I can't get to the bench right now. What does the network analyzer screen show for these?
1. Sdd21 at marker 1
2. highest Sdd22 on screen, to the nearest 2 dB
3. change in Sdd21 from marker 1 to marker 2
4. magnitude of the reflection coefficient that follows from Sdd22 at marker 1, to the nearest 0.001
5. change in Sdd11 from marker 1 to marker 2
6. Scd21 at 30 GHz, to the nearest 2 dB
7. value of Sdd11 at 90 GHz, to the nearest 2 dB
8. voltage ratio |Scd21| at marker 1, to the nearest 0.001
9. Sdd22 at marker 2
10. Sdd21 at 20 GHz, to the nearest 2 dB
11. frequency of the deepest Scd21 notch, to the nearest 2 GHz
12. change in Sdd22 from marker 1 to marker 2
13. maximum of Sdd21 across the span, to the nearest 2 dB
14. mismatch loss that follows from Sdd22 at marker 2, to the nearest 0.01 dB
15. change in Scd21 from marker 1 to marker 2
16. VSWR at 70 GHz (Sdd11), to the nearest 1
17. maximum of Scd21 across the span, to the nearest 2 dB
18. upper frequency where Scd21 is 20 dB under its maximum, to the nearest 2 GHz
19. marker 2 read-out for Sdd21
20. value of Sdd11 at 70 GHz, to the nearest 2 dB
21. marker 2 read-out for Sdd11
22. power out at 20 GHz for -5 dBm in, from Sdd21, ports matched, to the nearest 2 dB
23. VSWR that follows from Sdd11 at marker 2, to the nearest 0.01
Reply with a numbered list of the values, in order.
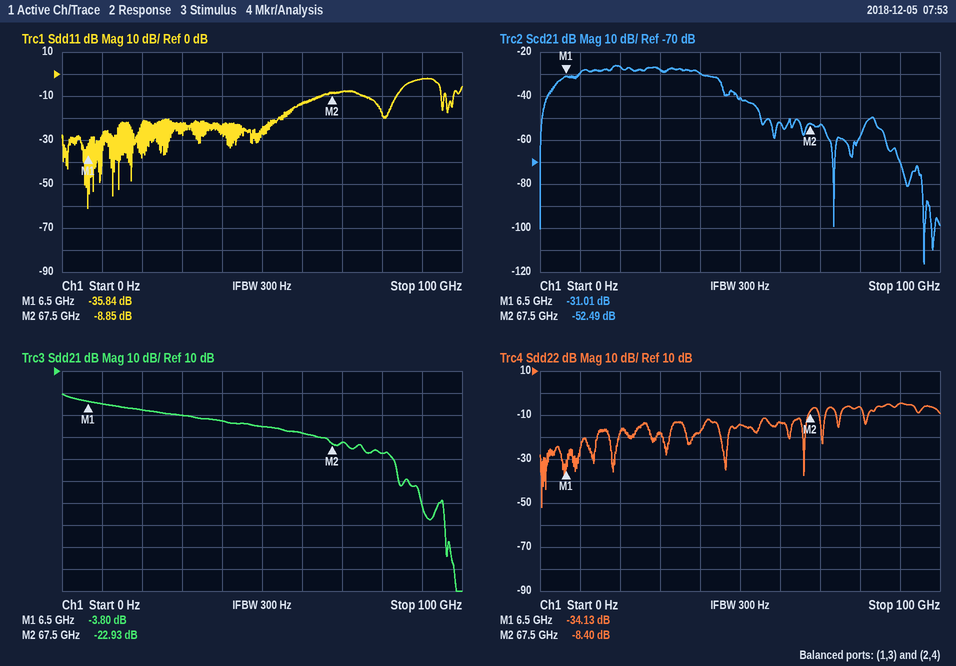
1. -3.80 dB
2. -4 dB
3. -19.13 dB
4. 0.020
5. 26.99 dB
6. -28 dB
7. -2 dB
8. 0.028
9. -8.40 dB
10. -8 dB
11. 96 GHz
12. 25.73 dB
13. 0 dB
14. 0.68 dB
15. -21.48 dB
16. 2
17. -26 dB
18. 54 GHz
19. -22.93 dB
20. -8 dB
21. -8.85 dB
22. -12 dBm
23. 2.13
